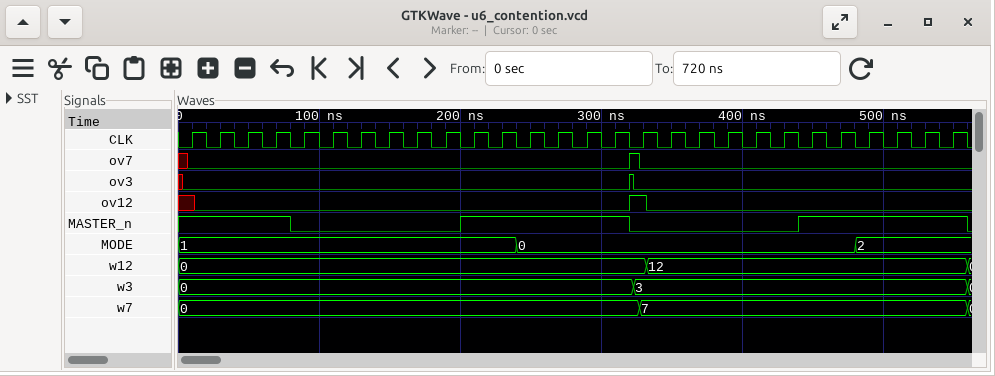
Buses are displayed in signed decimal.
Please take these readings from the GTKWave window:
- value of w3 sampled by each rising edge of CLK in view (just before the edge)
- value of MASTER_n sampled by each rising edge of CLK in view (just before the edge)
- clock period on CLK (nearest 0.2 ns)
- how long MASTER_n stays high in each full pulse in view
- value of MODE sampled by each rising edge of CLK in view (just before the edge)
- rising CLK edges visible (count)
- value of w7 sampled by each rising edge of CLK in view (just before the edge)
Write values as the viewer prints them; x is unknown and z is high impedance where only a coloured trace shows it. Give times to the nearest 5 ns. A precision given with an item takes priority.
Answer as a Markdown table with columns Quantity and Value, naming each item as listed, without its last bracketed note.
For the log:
| Quantity | Value |
|---|---|
| value of w3 sampled by each rising edge of CLK in view | 0, 0, 0, 0, 0, 0, 0, 0, 0, 0, 0, 0, 0, 0, 0, 0, 3, 3, 3, 3, 3, 3, 3, 3, 3, 3, 3, 3 |
| value of MASTER_n sampled by each rising edge of CLK in view | 1 1 1 1 0 0 0 0 0 0 1 1 1 1 1 1 0 0 0 0 0 0 1 1 1 1 1 1 |
| clock period on CLK | 20 ns |
| how long MASTER_n stays high in each full pulse in view | 120 ns, 120 ns |
| value of MODE sampled by each rising edge of CLK in view | 1, 1, 1, 1, 1, 1, 1, 1, 1, 1, 1, 1, 0, 0, 0, 0, 0, 0, 0, 0, 0, 0, 0, 0, 2, 2, 2, 2 |
| rising CLK edges visible | 28 |
| value of w7 sampled by each rising edge of CLK in view | 0, 0, 0, 0, 0, 0, 0, 0, 0, 0, 0, 0, 0, 0, 0, 0, 7, 7, 7, 7, 7, 7, 7, 7, 7, 7, 7, 7 |
